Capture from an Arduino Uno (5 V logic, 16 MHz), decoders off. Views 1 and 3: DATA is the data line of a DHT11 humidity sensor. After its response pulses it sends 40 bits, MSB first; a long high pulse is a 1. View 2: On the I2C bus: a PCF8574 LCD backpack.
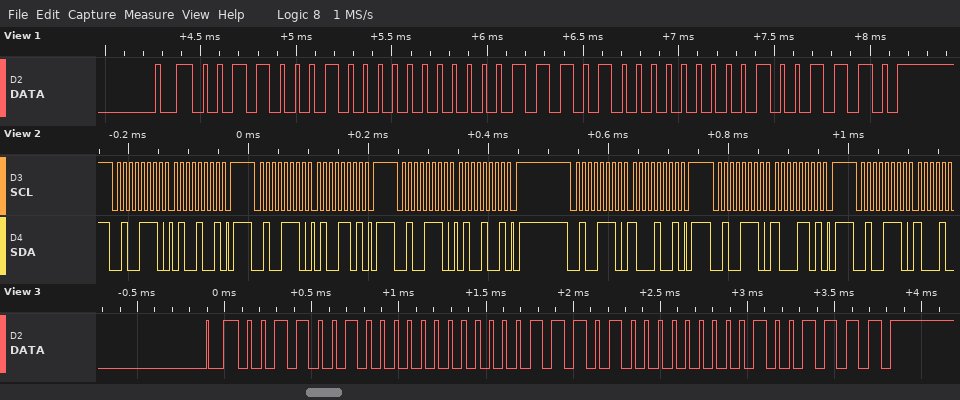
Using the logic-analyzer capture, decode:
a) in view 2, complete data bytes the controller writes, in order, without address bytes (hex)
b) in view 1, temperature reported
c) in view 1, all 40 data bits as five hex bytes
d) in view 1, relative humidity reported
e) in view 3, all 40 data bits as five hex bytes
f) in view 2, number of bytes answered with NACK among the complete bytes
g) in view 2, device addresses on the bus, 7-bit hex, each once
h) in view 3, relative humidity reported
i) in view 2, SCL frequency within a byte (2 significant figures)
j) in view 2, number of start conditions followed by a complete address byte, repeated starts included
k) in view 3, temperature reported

49 4D 49 89 8D
29.0 °C
31 00 1D 00 4E
49 %
32 00 1D 00 4F
0
0x27
50 %
100 kHz
6
29.0 °C
